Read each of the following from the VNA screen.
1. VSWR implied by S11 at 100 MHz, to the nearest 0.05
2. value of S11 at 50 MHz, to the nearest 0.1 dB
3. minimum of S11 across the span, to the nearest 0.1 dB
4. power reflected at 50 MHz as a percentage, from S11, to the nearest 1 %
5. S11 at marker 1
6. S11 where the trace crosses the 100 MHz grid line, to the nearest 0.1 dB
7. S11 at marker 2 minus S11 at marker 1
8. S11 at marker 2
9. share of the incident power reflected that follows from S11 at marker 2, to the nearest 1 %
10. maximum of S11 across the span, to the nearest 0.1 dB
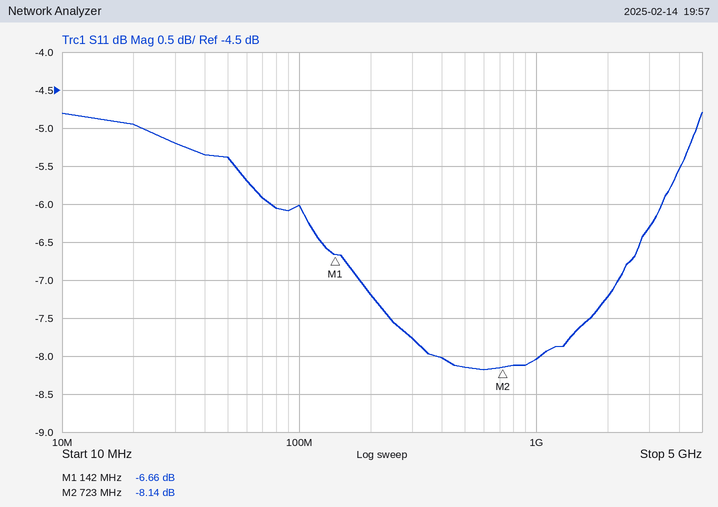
3.00
-5.4 dB
-8.2 dB
29 %
-6.66 dB
-6.0 dB
-1.48 dB
-8.14 dB
15 %
-4.8 dB
